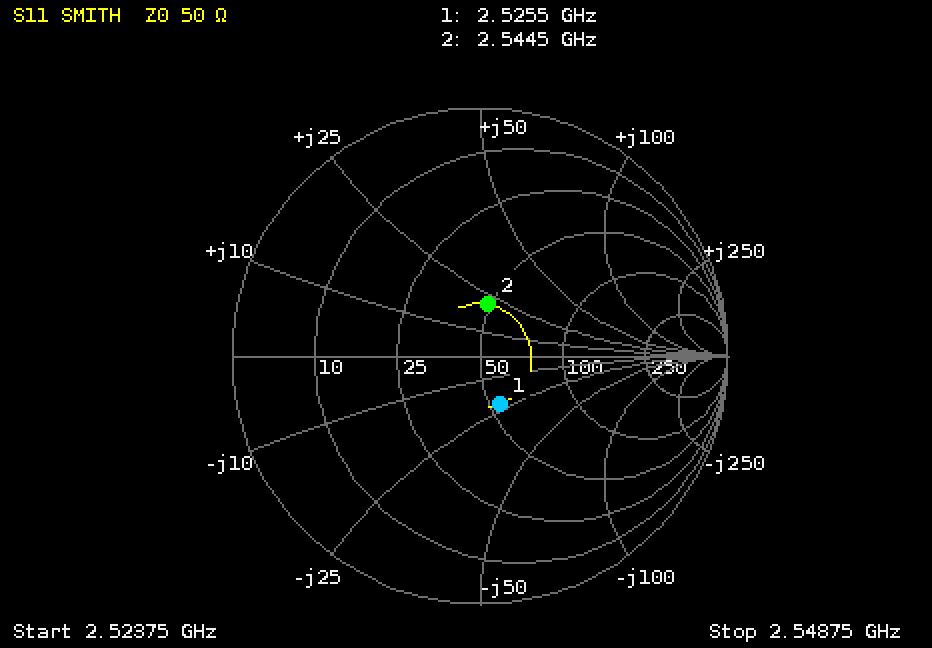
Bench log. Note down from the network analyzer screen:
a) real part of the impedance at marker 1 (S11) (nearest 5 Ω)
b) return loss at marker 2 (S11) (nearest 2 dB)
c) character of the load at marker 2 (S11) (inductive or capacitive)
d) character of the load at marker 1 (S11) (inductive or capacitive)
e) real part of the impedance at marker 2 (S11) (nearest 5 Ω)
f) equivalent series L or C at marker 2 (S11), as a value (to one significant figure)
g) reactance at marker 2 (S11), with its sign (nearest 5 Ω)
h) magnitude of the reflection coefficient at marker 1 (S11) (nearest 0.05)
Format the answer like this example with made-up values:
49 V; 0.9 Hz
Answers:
55 Ω; 14 dB; inductive; capacitive; 50 Ω; 1 nH; +20 Ω; 0.20
